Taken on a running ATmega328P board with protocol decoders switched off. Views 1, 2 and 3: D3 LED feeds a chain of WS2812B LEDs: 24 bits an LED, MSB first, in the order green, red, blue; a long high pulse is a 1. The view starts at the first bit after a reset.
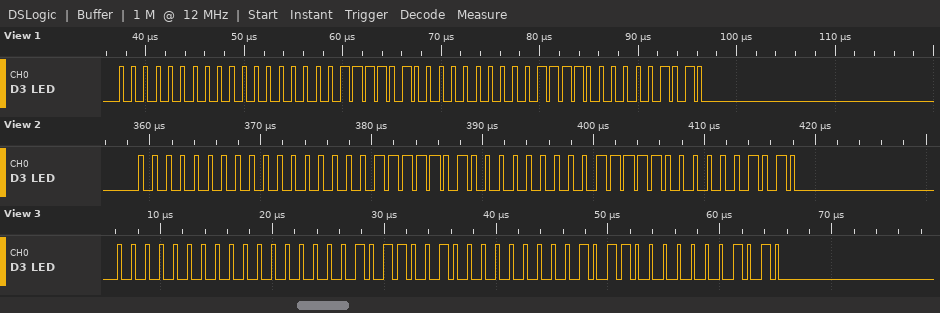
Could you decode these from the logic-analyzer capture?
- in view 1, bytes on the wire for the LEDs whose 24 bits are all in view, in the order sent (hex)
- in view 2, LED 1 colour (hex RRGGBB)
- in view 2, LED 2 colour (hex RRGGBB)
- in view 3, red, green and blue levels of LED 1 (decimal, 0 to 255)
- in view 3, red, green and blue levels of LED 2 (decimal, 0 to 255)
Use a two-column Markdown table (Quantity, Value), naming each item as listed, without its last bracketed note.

| Quantity | Value |
|---|---|
| in view 1, bytes on the wire for the LEDs whose 24 bits are all in view, in the order sent | 00 00 3D 00 3C 0A |
| in view 2, LED 1 colour | #00007D |
| in view 2, LED 2 colour | #7C000A |
| in view 3, red, green and blue levels of LED 1 | 0, 0, 89 |
| in view 3, red, green and blue levels of LED 2 | 88, 0, 10 |
